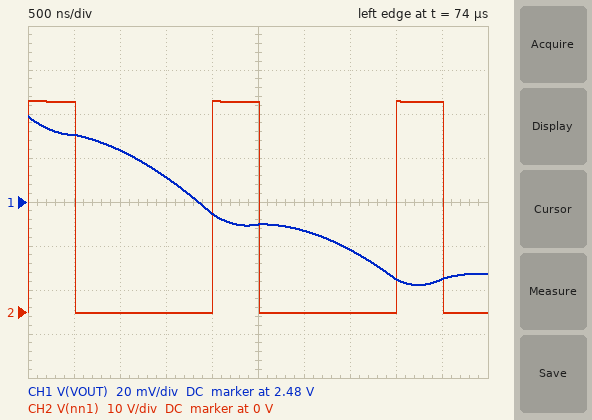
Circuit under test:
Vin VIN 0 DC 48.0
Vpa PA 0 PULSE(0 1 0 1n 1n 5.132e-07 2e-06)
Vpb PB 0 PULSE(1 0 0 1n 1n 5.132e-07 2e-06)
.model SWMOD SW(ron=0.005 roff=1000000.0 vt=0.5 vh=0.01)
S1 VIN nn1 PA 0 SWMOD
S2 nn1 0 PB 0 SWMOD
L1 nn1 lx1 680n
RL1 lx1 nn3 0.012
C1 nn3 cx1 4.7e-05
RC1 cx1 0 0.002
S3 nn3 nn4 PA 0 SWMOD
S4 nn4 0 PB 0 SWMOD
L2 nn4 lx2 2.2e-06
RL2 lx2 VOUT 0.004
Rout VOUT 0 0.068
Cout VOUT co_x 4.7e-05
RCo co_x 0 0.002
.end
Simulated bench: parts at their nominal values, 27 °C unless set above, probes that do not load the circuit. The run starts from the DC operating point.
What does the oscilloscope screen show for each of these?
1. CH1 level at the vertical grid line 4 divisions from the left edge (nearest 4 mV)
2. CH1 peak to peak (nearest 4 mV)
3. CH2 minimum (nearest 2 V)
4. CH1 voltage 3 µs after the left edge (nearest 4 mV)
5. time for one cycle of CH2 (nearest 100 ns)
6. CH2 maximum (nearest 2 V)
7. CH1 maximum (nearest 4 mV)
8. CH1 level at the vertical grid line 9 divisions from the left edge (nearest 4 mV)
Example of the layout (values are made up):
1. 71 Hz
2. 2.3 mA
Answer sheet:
1. 2.476 V
2. 76 mV
3. 0 V
4. 2.468 V
5. 2.0 µs
6. 48 V
7. 2.520 V
8. 2.444 V
